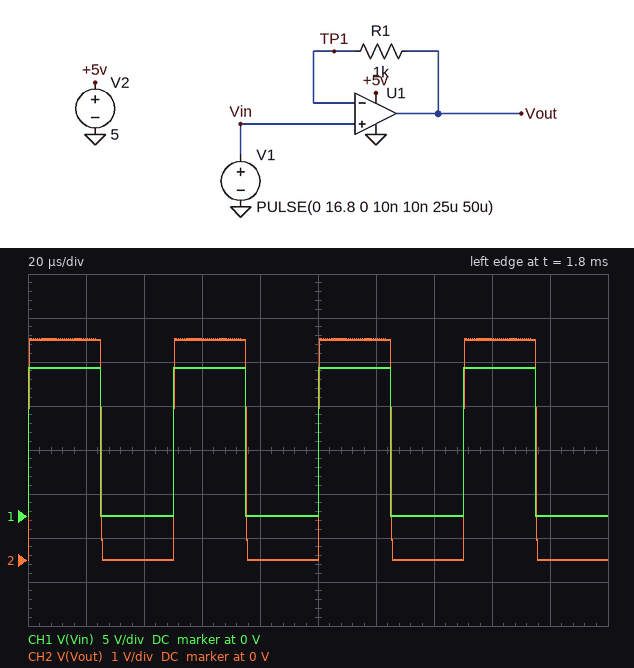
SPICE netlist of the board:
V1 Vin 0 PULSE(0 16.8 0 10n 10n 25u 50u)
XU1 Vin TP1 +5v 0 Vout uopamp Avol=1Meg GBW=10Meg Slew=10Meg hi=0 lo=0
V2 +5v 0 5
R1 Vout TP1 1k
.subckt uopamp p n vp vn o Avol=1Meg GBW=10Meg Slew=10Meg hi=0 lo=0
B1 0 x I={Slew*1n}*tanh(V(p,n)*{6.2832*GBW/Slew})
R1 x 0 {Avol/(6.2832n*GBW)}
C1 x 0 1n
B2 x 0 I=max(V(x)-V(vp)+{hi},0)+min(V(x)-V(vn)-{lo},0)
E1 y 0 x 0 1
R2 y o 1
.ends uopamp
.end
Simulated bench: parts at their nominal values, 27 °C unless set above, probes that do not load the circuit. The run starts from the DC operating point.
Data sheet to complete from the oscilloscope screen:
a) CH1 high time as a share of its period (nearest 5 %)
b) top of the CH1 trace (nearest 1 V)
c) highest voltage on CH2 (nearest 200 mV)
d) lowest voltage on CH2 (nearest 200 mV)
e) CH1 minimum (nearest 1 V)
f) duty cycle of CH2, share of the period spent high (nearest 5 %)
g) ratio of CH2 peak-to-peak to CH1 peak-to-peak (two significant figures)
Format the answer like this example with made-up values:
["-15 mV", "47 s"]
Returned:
["50 %", "17 V", "5.0 V", "0 V", "0 V", "50 %", "0.30"]
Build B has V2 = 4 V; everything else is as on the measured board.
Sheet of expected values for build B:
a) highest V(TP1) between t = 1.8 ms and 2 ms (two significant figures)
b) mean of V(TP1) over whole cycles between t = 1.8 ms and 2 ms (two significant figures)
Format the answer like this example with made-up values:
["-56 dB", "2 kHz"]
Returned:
["4.0 V", "2.0 V"]
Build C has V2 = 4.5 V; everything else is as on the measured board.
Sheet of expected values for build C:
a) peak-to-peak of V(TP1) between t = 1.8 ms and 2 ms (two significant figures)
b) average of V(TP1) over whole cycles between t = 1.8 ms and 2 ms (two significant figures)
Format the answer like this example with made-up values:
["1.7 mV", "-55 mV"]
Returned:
["4.5 V", "2.3 V"]
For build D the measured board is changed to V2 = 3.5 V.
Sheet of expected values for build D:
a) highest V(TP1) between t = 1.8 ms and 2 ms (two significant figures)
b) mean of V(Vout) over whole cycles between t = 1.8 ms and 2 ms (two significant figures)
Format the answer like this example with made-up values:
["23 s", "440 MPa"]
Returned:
["3.5 V", "1.8 V"]
